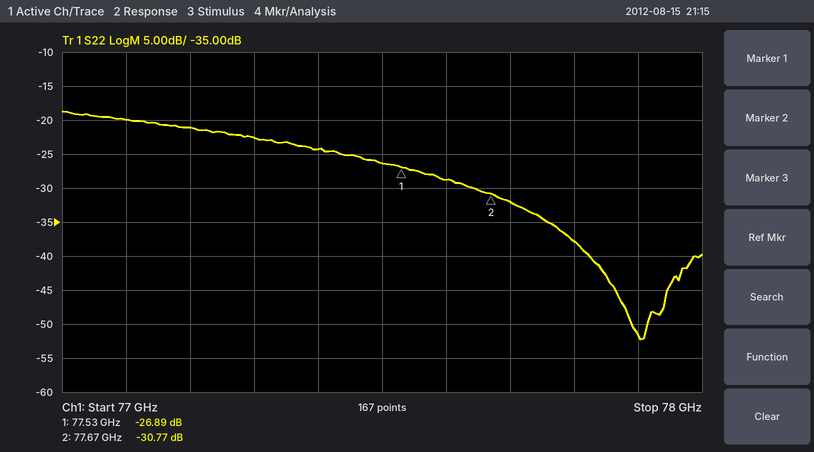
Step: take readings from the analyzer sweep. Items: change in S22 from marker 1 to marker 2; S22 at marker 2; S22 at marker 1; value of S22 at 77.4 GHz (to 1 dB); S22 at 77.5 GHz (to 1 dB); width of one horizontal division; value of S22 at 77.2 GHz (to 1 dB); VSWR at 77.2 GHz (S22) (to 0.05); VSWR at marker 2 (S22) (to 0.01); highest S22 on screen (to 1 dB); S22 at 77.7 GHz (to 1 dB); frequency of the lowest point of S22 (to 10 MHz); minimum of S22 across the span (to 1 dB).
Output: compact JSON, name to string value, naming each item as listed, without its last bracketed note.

{"change in S22 from marker 1 to marker 2": "-3.88 dB", "S22 at marker 2": "-30.77 dB", "S22 at marker 1": "-26.89 dB", "value of S22 at 77.4 GHz": "-24 dB", "S22 at 77.5 GHz": "-26 dB", "width of one horizontal division": "100 MHz", "value of S22 at 77.2 GHz": "-21 dB", "VSWR at 77.2 GHz (S22)": "1.20", "VSWR at marker 2 (S22)": "1.06", "highest S22 on screen": "-19 dB", "S22 at 77.7 GHz": "-32 dB", "frequency of the lowest point of S22": "77.90 GHz", "minimum of S22 across the span": "-52 dB"}
